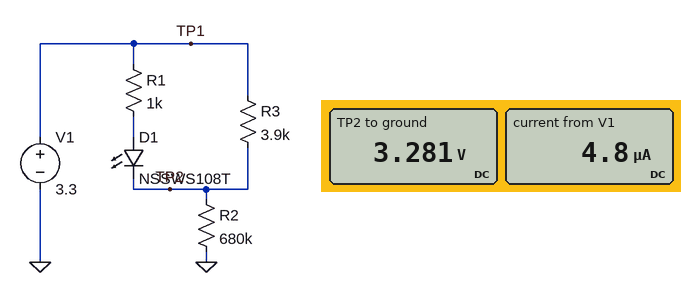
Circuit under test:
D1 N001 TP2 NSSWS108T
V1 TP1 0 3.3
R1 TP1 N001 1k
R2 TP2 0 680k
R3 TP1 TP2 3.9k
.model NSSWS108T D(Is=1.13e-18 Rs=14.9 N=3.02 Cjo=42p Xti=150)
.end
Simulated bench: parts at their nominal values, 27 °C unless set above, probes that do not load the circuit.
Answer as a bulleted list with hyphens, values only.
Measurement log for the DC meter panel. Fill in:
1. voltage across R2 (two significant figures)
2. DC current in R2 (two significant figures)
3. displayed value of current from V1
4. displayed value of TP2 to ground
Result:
- 3.3 V
- 4.8 µA
- 4.8 µA
- 3.281 V
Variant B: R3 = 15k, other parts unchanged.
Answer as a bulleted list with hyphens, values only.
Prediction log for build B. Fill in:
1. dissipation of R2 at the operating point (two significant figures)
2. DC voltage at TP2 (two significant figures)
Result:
- 15 µW
- 3.2 V
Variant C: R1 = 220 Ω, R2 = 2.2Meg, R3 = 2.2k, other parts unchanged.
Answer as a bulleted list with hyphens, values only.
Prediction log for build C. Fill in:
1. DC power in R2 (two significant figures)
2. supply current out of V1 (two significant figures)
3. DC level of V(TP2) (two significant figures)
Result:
- 4.9 µW
- 1.5 µA
- 3.3 V
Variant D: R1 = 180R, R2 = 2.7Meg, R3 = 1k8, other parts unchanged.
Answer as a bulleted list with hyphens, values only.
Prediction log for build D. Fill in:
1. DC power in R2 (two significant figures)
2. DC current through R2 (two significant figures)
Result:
- 4.0 µW
- 1.2 µA
